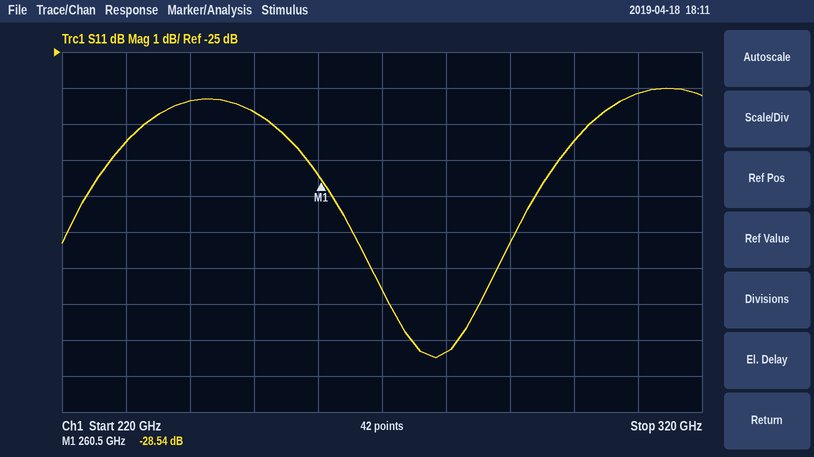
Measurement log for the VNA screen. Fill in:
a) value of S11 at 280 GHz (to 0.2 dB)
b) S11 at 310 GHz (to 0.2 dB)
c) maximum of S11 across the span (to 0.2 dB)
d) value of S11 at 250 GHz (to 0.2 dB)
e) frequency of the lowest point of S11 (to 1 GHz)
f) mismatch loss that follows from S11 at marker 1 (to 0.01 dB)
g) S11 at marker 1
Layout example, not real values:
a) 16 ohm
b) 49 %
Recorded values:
a) -33.4 dB
b) -26.2 dB
c) -26.0 dB
d) -26.6 dB
e) 278 GHz
f) 0.01 dB
g) -28.54 dB
